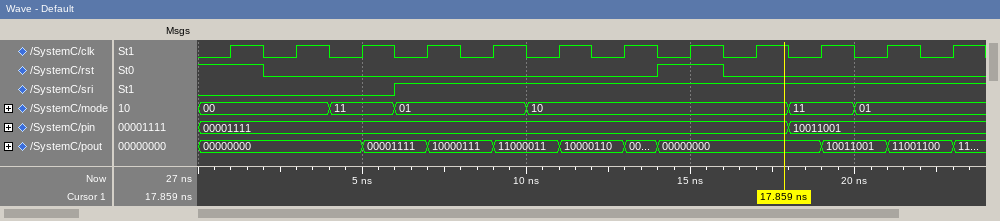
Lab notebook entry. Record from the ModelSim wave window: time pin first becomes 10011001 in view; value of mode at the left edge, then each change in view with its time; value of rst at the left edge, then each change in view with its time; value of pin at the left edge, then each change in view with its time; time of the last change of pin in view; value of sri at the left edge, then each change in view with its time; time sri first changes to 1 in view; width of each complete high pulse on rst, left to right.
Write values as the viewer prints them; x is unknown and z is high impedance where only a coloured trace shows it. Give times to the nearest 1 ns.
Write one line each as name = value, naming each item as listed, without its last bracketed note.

time pin first becomes 10011001 in view = 18 ns
value of mode at the left edge, then each change in view with its time = 00, 11 at 4 ns, 01 at 6 ns, 10 at 10 ns, 11 at 18 ns, 01 at 20 ns
value of rst at the left edge, then each change in view with its time = 1, 0 at 2 ns, 1 at 14 ns, 0 at 16 ns
value of pin at the left edge, then each change in view with its time = 00001111, 10011001 at 18 ns
time of the last change of pin in view = 18 ns
value of sri at the left edge, then each change in view with its time = 0, 1 at 6 ns
time sri first changes to 1 in view = 6 ns
width of each complete high pulse on rst, left to right = 2 ns
